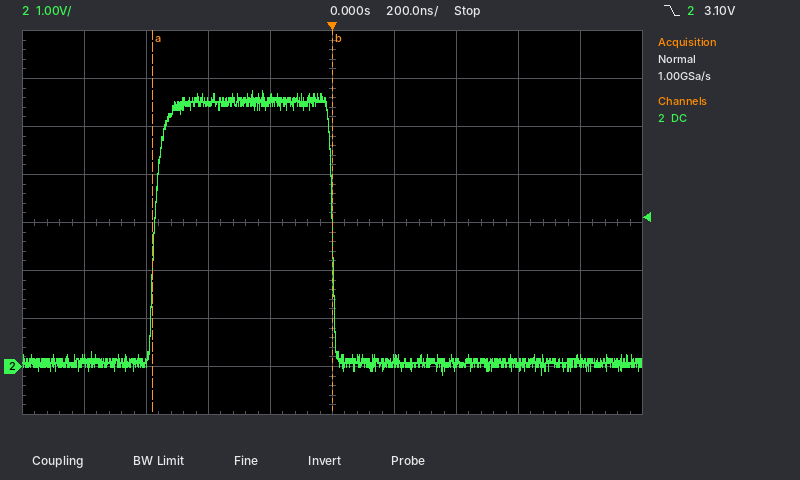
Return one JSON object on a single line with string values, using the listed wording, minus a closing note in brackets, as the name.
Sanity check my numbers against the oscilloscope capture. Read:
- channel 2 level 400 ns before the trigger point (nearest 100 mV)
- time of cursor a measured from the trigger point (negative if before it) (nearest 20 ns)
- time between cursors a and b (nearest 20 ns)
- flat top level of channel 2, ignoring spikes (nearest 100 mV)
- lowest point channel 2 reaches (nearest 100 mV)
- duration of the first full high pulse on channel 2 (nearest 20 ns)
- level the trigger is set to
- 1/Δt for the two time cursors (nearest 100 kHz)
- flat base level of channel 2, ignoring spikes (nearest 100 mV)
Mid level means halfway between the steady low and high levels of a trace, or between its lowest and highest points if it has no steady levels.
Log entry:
{"channel 2 level 400 ns before the trigger point": "5.5 V", "time of cursor a measured from the trigger point (negative if before it)": "-580 ns", "time between cursors a and b": "580 ns", "flat top level of channel 2, ignoring spikes": "5.5 V", "lowest point channel 2 reaches": "-200 mV", "duration of the first full high pulse on channel 2": "580 ns", "level the trigger is set to": "3.10 V", "1/Δt for the two time cursors": "1.7 MHz", "flat base level of channel 2, ignoring spikes": "100 mV"}
